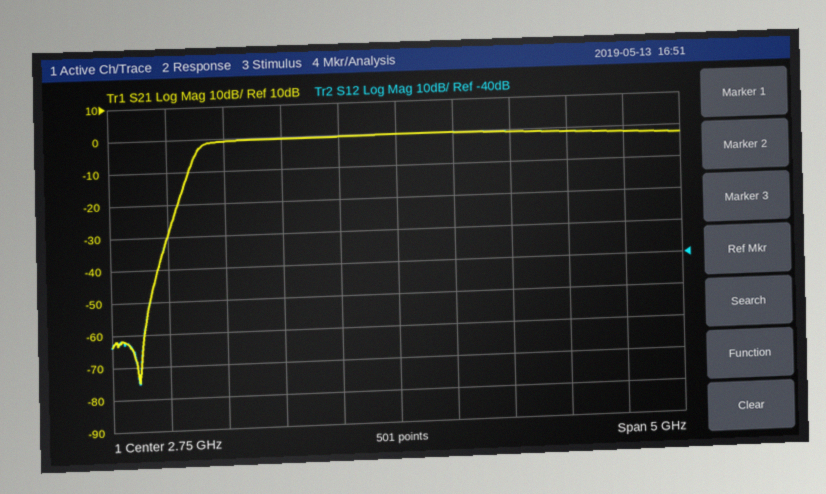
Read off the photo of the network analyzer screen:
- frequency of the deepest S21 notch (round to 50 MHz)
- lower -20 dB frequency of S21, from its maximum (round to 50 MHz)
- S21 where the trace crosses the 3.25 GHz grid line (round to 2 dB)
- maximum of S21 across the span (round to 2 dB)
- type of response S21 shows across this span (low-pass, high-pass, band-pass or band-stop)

500 MHz
850 MHz
0 dB
0 dB
high-pass
